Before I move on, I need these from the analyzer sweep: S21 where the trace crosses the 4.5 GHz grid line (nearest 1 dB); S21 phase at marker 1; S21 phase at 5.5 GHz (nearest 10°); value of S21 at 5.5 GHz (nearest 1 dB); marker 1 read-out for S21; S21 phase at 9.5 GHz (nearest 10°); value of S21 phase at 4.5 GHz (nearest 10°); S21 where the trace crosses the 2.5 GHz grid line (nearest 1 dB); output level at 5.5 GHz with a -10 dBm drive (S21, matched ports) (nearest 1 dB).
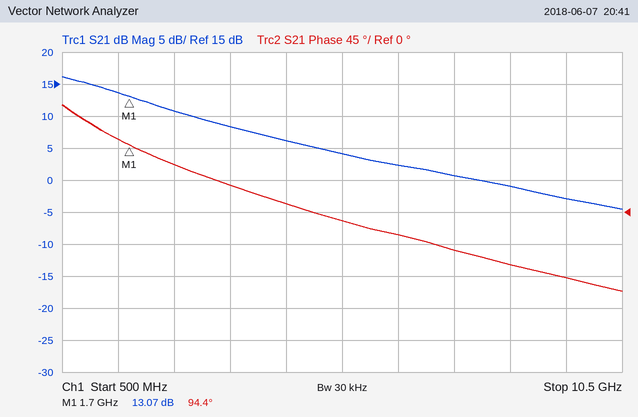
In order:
6 dB
94.4°
-10°
4 dB
13.07 dB
-90°
10°
11 dB
-6 dBm
